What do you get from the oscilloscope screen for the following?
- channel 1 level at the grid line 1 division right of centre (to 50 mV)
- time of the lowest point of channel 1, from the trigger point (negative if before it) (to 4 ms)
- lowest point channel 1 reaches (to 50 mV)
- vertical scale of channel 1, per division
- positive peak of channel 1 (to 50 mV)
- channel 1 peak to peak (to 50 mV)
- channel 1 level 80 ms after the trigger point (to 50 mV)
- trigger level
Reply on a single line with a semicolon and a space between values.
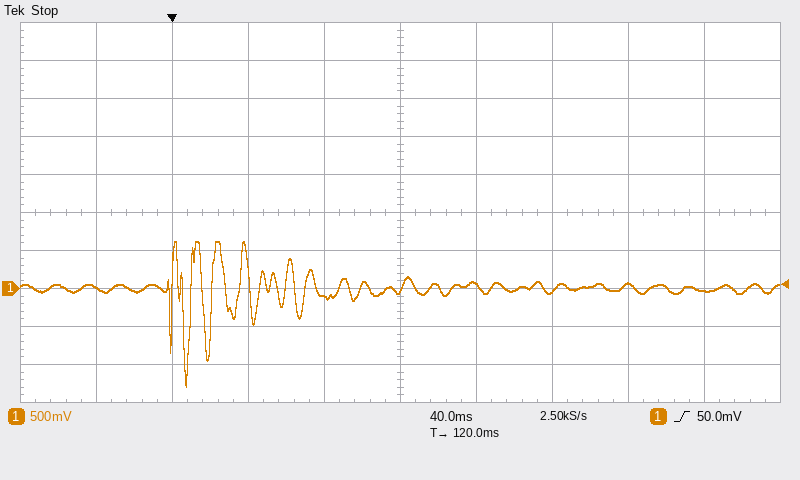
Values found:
50 mV; +8 ms; -1.30 V; 500 mV; 600 mV; 1.90 V; -100 mV; 50.0 mV
